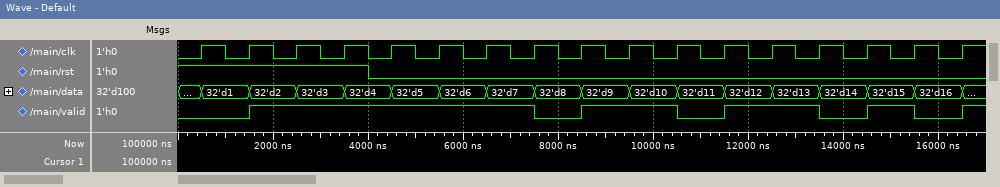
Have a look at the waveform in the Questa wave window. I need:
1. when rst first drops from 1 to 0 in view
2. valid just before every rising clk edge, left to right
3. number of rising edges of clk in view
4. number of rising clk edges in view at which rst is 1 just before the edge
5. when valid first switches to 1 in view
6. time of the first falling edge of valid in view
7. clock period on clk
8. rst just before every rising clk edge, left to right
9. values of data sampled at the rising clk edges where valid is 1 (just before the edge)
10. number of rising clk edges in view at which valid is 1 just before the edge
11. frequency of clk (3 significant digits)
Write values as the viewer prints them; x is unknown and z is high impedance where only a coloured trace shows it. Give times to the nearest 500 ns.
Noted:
4000 ns
0 0 1 1 1 1 1 1 0 1 1 0 1 1 0 1 0
17
4
1500 ns
7500 ns
1000 ns
1 1 1 1 0 0 0 0 0 0 0 0 0 0 0 0 0
32'd2, 32'd3, 32'd4, 32'd5, 32'd6, 32'd7, 32'd9, 32'd10, 32'd12, 32'd13, 32'd15
11
1.00 MHz
